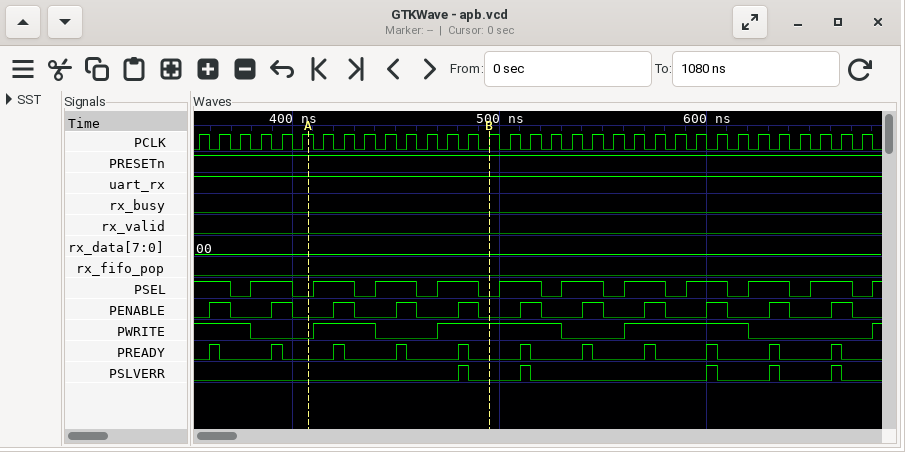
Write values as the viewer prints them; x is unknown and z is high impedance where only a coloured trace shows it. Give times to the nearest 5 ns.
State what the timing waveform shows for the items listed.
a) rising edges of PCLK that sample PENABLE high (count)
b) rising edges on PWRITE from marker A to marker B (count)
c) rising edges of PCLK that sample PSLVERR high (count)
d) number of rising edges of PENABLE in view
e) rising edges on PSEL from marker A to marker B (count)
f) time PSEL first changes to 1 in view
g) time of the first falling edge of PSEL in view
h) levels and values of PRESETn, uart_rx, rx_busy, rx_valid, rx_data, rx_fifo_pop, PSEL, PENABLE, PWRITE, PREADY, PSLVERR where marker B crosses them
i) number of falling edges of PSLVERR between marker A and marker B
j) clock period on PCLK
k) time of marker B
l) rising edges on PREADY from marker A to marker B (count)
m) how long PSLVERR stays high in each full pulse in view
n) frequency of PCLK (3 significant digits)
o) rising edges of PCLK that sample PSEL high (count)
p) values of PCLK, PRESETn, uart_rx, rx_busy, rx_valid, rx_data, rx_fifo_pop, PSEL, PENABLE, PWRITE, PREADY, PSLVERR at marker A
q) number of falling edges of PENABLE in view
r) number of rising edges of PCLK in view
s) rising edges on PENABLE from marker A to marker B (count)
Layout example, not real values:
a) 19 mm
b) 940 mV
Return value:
a) 11
b) 2
c) 5
d) 11
e) 3
f) 380 ns
g) 370 ns
h) PRESETn=1, uart_rx=1, rx_busy=0, rx_valid=0, rx_data=00, rx_fifo_pop=0, PSEL=0, PENABLE=0, PWRITE=1, PREADY=0, PSLVERR=0
i) 1
j) 10 ns
k) 495 ns
l) 3
m) 5 ns, 5 ns, 5 ns, 5 ns, 5 ns
n) 100 MHz
o) 22
p) PCLK=1, PRESETn=1, uart_rx=1, rx_busy=0, rx_valid=0, rx_data=00, rx_fifo_pop=0, PSEL=0, PENABLE=0, PWRITE=0, PREADY=0, PSLVERR=0
q) 11
r) 33
s) 3
